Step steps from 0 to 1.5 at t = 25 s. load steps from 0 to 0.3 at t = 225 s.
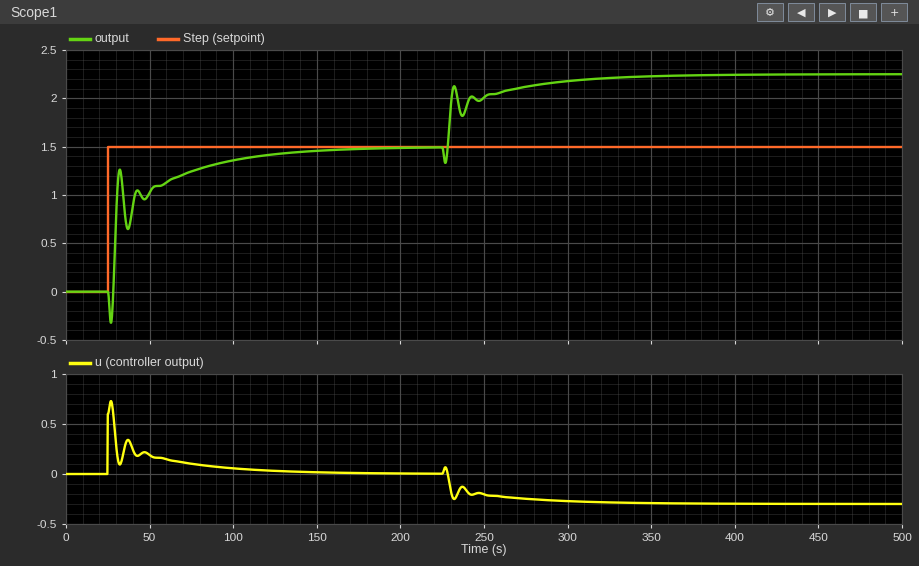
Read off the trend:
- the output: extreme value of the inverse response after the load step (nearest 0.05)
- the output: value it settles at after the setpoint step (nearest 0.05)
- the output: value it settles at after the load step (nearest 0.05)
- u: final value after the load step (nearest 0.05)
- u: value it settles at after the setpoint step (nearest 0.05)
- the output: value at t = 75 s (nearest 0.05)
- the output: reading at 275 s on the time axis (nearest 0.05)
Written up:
1.35
1.50
2.25
-0.30
0.00
1.25
2.10
